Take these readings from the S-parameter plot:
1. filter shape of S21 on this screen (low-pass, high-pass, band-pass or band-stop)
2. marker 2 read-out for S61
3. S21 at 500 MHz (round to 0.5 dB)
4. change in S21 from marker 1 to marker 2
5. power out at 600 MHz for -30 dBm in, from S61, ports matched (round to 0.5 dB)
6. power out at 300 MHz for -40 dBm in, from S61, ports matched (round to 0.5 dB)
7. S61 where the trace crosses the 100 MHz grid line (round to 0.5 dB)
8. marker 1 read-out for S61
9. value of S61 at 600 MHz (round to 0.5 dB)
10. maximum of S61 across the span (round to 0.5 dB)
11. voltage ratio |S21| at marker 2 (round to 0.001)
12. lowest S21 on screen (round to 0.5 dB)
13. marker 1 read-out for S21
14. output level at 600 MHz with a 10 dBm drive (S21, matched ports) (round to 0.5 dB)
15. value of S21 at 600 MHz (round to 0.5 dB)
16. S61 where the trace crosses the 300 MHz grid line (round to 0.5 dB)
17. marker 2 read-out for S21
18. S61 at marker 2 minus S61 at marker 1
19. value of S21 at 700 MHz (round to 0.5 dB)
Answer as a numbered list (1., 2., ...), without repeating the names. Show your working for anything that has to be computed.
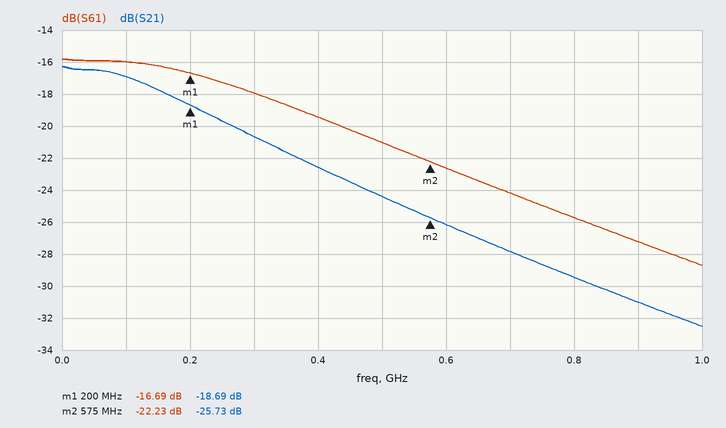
1. low-pass
2. -22.23 dB
3. -24.5 dB
4. -25.73 − (-18.69) = -7.04 dB
5. -30 dBm + (-22.5 dB) = -52.5 dBm
6. -40 dBm + (-18.0 dB) = -58.0 dBm
7. -16.0 dB
8. -16.69 dB
9. -22.5 dB
10. -16.0 dB
11. 10^(-25.73/20) ≈ 0.052
12. -32.5 dB
13. -18.69 dB
14. 10 dBm + (-26.0 dB) = -16.0 dBm
15. -26.0 dB
16. -18.0 dB
17. -25.73 dB
18. -22.23 − (-16.69) = -5.54 dB
19. -28.0 dB
